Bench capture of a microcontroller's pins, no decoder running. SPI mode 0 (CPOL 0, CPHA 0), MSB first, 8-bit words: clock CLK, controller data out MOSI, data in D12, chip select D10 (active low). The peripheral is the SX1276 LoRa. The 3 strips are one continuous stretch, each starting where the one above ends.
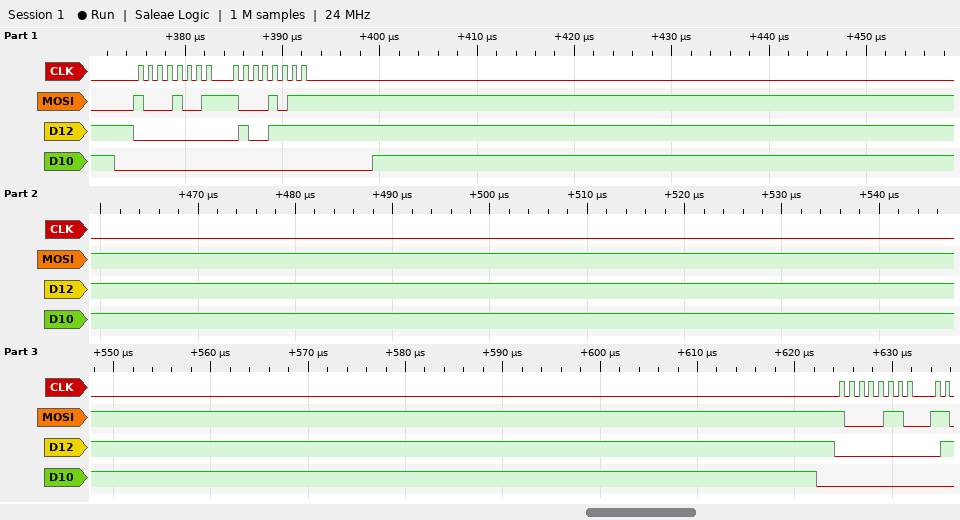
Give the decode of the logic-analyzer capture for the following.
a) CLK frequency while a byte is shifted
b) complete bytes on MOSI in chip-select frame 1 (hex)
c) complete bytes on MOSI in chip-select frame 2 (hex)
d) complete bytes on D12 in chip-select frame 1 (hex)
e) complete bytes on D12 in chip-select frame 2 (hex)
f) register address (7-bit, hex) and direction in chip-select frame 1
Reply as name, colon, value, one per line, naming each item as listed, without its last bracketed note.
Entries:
CLK frequency while a byte is shifted: 1 MHz
complete bytes on MOSI in chip-select frame 1: 89 8B
complete bytes on MOSI in chip-select frame 2: 86
complete bytes on D12 in chip-select frame 1: 00 4F
complete bytes on D12 in chip-select frame 2: 00
register address (7-bit, hex) and direction in chip-select frame 1: 0x09 write
